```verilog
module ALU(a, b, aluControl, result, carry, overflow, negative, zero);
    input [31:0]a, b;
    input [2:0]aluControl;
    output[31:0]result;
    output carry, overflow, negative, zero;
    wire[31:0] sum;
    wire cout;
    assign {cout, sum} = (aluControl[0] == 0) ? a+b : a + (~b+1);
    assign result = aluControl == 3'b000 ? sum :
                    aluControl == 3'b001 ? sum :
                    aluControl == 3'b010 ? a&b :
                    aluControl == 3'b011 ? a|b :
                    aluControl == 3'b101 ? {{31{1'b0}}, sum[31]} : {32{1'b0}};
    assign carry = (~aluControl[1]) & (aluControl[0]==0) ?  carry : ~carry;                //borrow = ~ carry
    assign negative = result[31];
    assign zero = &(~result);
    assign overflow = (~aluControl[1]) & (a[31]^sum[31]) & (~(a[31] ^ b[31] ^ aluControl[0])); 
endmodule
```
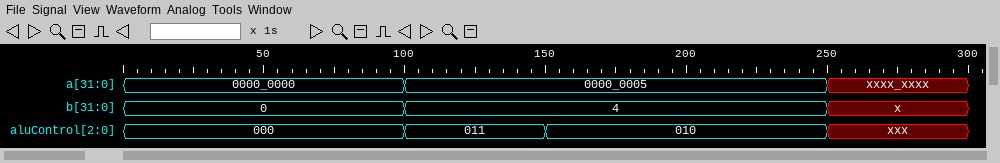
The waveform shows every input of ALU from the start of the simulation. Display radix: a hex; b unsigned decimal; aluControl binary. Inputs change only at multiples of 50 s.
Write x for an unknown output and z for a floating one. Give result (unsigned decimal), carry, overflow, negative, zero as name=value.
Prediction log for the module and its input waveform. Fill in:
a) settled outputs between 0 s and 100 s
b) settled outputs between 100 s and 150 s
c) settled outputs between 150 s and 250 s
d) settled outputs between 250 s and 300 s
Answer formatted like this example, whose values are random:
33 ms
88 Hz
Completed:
result=0, carry=z, overflow=0, negative=0, zero=1
result=5, carry=z, overflow=0, negative=0, zero=0
result=4, carry=z, overflow=0, negative=0, zero=0
result=x, carry=z, overflow=x, negative=x, zero=x
